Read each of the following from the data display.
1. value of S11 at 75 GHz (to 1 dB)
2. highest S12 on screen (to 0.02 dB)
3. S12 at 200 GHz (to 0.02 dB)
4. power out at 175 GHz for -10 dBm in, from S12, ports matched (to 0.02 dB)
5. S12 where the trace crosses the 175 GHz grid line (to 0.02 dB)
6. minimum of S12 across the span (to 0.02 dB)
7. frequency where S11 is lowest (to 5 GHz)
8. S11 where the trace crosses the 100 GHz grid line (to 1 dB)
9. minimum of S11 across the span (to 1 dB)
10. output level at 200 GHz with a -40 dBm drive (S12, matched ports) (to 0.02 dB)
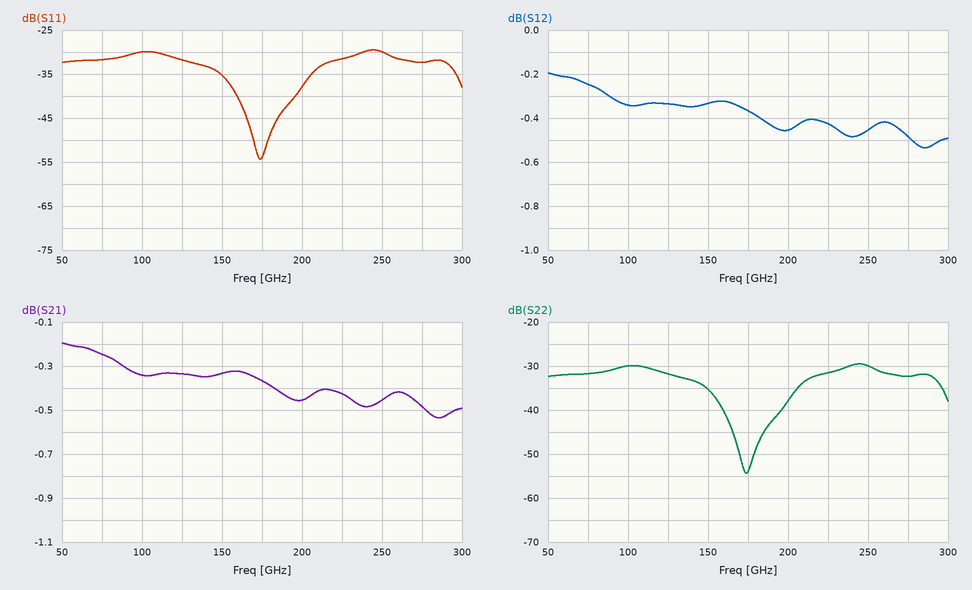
-32 dB
-0.20 dB
-0.46 dB
-10.36 dBm
-0.36 dB
-0.54 dB
175 GHz
-30 dB
-54 dB
-40.46 dBm
